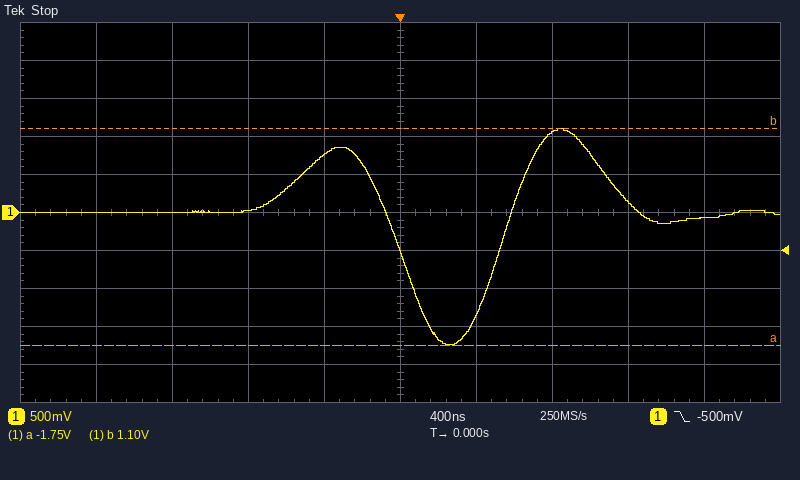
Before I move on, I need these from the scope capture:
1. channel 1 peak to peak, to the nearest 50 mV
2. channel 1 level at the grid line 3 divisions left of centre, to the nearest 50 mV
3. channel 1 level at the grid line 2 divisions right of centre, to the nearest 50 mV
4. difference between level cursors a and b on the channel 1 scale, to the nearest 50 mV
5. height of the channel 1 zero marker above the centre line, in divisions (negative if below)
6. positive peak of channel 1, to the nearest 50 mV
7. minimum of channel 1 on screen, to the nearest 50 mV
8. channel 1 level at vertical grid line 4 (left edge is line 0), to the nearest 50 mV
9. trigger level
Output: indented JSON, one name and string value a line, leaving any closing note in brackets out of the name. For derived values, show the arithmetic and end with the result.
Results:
{
  "channel 1 peak to peak, to the nearest 50 mV": "1.10 V − (-1.75 V) = 2.85 V",
  "channel 1 level at the grid line 3 divisions left of centre, to the nearest 50 mV": "0 mV",
  "channel 1 level at the grid line 2 divisions right of centre, to the nearest 50 mV": "1.05 V",
  "difference between level cursors a and b on the channel 1 scale, to the nearest 50 mV": "2.85 V",
  "height of the channel 1 zero marker above the centre line, in divisions": "0.0 div",
  "positive peak of channel 1, to the nearest 50 mV": "1.10 V",
  "minimum of channel 1 on screen, to the nearest 50 mV": "-1.75 V",
  "channel 1 level at vertical grid line 4 (left edge is line 0), to the nearest 50 mV": "750 mV",
  "trigger level": "-500 mV"
}
